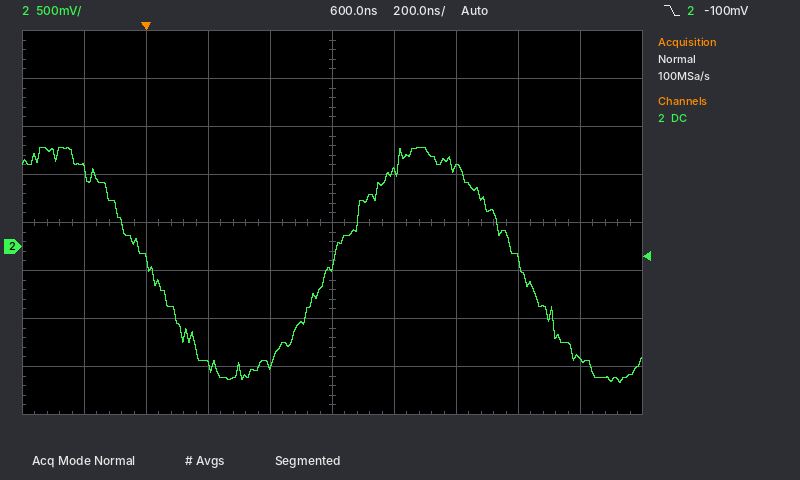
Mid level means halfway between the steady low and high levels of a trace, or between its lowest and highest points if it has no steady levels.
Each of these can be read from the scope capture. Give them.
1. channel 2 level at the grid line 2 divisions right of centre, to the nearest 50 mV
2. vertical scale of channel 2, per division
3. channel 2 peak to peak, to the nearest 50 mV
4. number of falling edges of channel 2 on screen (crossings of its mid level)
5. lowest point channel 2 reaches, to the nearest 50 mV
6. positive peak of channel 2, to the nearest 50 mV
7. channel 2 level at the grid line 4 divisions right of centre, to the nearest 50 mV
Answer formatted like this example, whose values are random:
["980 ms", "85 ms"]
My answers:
["800 mV", "500 mV", "2.45 V", "2", "-1.40 V", "1.05 V", "-1.15 V"]
